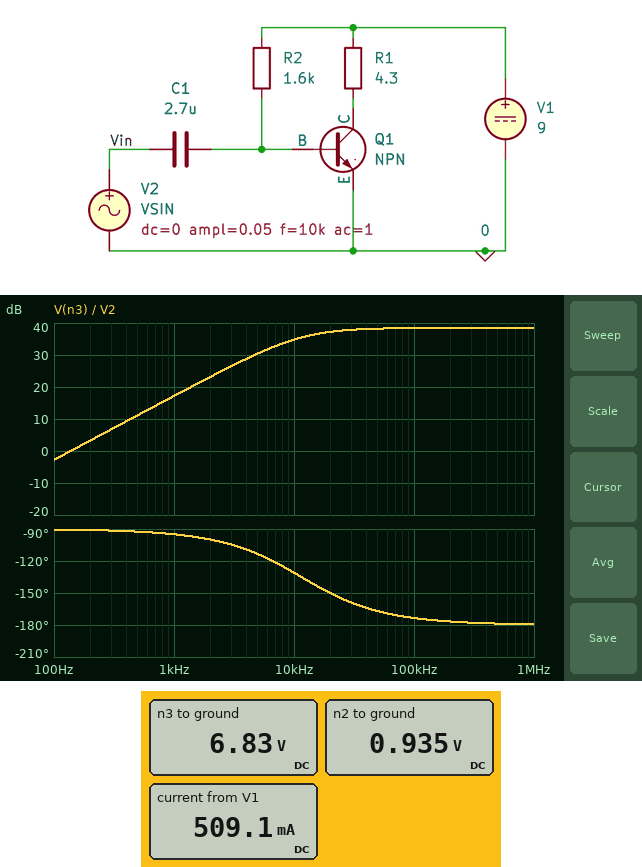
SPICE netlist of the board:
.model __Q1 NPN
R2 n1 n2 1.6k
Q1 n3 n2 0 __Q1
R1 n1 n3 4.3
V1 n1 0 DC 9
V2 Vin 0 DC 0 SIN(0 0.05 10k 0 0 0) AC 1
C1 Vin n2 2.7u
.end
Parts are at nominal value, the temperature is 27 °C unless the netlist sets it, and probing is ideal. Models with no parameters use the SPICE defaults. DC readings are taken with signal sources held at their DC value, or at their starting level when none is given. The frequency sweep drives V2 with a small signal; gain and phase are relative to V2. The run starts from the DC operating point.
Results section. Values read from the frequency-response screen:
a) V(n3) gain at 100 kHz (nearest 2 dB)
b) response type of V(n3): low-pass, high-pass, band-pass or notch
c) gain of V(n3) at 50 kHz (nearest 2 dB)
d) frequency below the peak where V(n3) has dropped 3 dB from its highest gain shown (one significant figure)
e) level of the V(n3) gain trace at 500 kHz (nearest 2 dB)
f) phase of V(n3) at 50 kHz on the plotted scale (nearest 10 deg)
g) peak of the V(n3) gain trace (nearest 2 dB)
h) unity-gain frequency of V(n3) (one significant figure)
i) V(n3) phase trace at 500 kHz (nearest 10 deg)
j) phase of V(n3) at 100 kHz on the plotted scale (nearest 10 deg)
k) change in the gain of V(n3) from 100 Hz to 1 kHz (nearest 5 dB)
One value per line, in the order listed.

38 dB
high-pass
38 dB
10 kHz
38 dB
-170 deg
38 dB
100 Hz
-180 deg
-170 deg
20 dB
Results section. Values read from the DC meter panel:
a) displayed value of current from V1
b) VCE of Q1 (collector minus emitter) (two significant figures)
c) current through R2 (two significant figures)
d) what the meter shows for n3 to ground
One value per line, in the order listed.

509.1 mA
6.8 V
5.0 mA
6.83 V
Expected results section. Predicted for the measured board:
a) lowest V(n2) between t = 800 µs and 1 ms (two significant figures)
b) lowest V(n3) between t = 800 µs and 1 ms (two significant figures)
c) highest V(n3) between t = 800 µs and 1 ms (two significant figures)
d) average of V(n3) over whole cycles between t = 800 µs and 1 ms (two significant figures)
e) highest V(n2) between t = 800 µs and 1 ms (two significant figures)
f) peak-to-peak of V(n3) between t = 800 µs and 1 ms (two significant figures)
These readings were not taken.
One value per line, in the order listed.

890 mV
3.8 V
8.7 V
6.8 V
960 mV
4.9 V
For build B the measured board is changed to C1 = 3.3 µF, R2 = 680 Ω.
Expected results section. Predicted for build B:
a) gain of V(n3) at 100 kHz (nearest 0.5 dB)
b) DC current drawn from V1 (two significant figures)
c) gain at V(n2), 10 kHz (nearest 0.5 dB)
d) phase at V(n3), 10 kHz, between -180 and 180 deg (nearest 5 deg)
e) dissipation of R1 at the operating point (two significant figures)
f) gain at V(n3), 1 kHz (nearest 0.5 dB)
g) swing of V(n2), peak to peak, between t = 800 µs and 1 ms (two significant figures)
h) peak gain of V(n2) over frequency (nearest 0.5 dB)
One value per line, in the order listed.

45.5 dB
1.2 A
-7.5 dB
-115 deg
6.0 W
19.0 dB
44 mV
0 dB
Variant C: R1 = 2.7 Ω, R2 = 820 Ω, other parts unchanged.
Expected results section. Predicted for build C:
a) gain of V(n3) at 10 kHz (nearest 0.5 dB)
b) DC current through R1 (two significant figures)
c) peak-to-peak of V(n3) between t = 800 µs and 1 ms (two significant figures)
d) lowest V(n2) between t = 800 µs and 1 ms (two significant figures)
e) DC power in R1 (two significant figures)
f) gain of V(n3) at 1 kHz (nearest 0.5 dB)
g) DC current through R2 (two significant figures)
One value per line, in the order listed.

32.5 dB
980 mA
4.0 V
920 mV
2.6 W
13.0 dB
9.8 mA
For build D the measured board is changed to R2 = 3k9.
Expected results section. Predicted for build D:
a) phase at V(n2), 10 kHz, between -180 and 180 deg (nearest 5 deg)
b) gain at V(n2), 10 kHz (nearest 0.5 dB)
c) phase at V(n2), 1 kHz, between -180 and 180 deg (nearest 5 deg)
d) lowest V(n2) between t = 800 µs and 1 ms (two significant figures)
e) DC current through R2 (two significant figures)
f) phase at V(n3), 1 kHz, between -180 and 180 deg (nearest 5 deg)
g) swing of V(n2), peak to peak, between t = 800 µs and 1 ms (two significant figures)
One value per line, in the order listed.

25 deg
-1.0 dB
80 deg
850 mV
2.1 mA
-100 deg
93 mV
